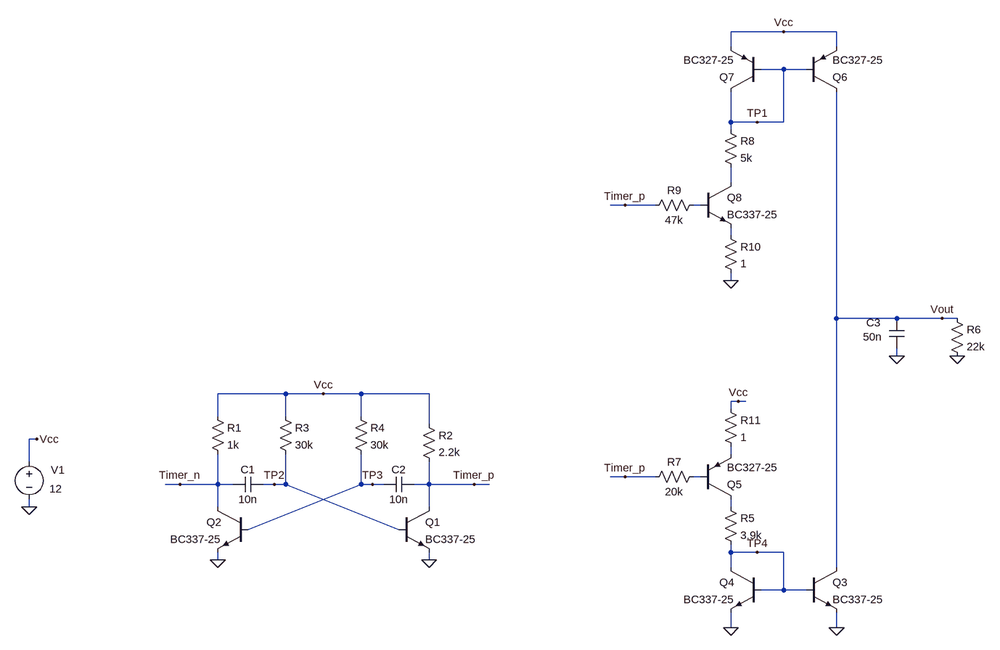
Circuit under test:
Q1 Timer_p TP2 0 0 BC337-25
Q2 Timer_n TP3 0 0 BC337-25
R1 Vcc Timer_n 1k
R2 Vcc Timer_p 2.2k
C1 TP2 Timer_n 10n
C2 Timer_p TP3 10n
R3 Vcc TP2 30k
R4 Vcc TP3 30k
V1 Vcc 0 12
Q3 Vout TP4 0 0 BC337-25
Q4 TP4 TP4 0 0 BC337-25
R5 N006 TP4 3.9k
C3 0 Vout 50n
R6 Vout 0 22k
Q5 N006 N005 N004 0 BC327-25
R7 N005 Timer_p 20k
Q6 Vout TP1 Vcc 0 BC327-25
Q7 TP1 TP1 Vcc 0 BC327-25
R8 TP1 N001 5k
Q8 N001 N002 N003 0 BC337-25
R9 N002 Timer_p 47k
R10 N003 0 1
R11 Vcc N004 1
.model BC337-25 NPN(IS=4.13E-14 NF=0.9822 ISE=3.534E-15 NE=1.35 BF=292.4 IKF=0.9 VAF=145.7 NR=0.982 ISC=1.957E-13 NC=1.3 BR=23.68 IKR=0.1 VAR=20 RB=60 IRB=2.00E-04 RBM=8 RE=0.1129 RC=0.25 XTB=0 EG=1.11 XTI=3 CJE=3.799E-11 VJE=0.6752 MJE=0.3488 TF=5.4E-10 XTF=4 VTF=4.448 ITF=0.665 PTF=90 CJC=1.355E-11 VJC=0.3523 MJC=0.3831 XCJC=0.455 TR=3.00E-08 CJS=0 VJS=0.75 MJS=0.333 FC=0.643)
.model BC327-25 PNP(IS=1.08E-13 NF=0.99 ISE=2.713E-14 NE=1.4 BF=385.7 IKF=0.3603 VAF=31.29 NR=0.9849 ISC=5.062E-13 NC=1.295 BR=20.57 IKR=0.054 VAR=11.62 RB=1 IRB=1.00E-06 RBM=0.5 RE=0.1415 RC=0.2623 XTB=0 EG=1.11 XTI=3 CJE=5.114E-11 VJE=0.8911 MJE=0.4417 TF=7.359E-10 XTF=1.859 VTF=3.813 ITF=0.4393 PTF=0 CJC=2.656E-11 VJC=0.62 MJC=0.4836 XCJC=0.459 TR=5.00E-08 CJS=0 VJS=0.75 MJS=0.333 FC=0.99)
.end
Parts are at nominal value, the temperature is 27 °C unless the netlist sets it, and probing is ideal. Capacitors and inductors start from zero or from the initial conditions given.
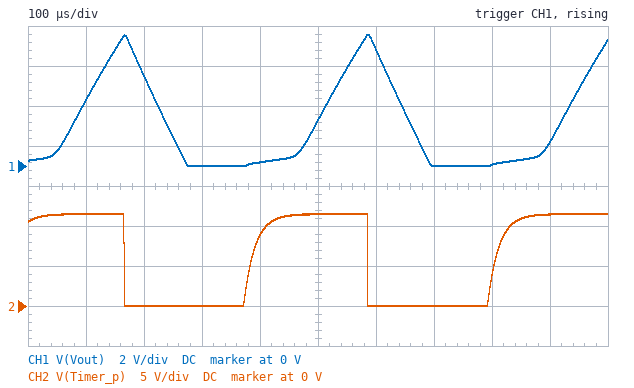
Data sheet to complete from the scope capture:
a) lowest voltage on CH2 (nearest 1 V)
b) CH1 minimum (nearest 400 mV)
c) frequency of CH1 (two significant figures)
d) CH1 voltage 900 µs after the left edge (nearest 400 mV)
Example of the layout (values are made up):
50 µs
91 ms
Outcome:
0 V
0 V
2.4 kHz
1.2 V
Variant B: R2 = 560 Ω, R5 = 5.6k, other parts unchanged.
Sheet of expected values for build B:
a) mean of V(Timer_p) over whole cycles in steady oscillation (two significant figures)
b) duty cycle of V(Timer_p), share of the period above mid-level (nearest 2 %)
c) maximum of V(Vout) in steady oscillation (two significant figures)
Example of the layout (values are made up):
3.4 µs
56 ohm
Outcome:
5.8 V
50 %
10 V
